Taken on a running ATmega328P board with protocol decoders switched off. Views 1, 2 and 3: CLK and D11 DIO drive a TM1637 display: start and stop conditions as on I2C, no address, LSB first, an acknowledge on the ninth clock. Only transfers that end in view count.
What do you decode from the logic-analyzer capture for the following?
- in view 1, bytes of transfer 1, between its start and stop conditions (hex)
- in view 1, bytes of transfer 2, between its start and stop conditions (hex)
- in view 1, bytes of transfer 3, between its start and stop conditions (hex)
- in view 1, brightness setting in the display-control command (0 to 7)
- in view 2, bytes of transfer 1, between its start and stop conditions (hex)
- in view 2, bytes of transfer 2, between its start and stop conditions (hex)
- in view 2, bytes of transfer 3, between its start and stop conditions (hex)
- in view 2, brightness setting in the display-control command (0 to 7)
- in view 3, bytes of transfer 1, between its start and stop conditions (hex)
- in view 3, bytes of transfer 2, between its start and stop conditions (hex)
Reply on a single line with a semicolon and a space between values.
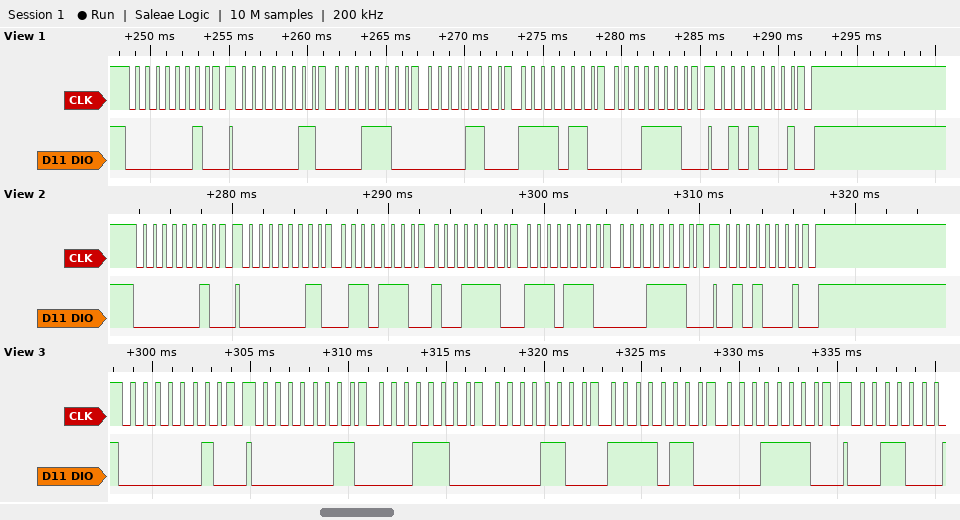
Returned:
40; C0 38 30 6F 78; 8A; 2; 40; C0 76 79 77 78; 8A; 2; 40; C0 38 30 6F 78
